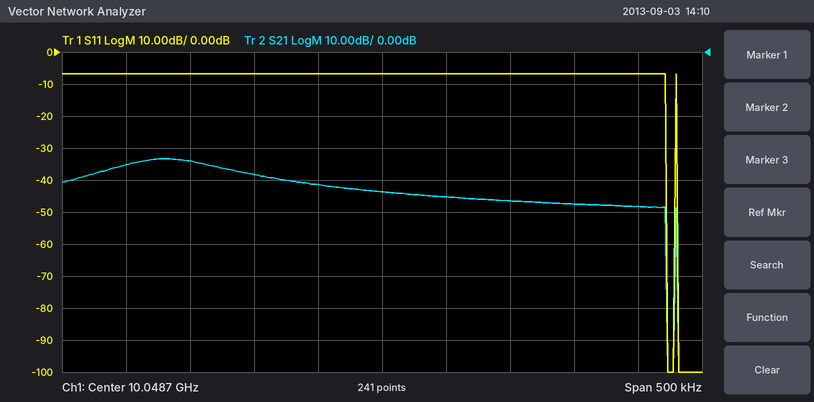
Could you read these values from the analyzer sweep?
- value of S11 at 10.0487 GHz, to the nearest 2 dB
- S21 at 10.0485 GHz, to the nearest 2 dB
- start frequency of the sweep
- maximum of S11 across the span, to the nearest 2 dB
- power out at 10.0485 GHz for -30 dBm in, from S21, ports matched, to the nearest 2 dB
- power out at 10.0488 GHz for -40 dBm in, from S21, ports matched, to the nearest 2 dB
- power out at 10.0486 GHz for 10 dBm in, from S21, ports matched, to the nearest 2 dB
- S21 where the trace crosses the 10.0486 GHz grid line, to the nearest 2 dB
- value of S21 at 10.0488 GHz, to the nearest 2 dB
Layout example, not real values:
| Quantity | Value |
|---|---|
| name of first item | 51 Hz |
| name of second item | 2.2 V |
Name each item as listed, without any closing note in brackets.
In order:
| Quantity | Value |
|---|---|
| value of S11 at 10.0487 GHz, to the nearest 2 dB | -6 dB |
| S21 at 10.0485 GHz, to the nearest 2 dB | -36 dB |
| start frequency of the sweep | 10.04845 GHz |
| maximum of S11 across the span, to the nearest 2 dB | -6 dB |
| power out at 10.0485 GHz for -30 dBm in, from S21, ports matched, to the nearest 2 dB | -66 dBm |
| power out at 10.0488 GHz for -40 dBm in, from S21, ports matched, to the nearest 2 dB | -86 dBm |
| power out at 10.0486 GHz for 10 dBm in, from S21, ports matched, to the nearest 2 dB | -28 dBm |
| S21 where the trace crosses the 10.0486 GHz grid line, to the nearest 2 dB | -38 dB |
| value of S21 at 10.0488 GHz, to the nearest 2 dB | -46 dB |
